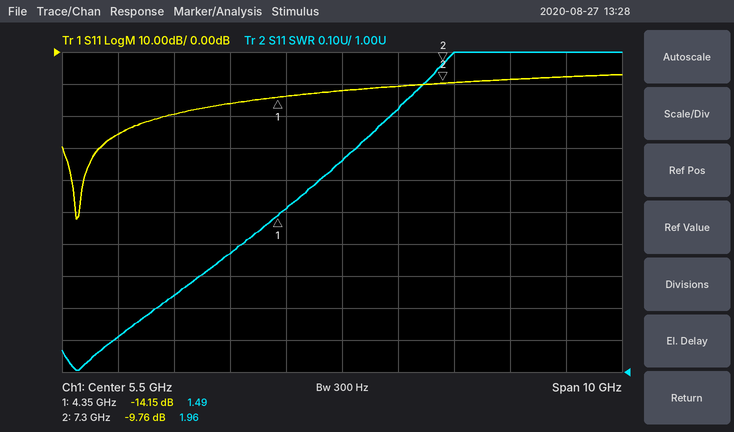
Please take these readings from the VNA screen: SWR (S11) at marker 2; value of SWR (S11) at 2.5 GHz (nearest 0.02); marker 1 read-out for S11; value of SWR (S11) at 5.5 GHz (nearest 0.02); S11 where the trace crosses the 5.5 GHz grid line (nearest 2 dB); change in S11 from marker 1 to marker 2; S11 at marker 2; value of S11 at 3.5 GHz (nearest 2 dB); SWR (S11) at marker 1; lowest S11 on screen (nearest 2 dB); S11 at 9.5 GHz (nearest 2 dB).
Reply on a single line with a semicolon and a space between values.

1.96; 1.24; -14.15 dB; 1.66; -12 dB; 4.39 dB; -9.76 dB; -16 dB; 1.49; -52 dB; -8 dB
